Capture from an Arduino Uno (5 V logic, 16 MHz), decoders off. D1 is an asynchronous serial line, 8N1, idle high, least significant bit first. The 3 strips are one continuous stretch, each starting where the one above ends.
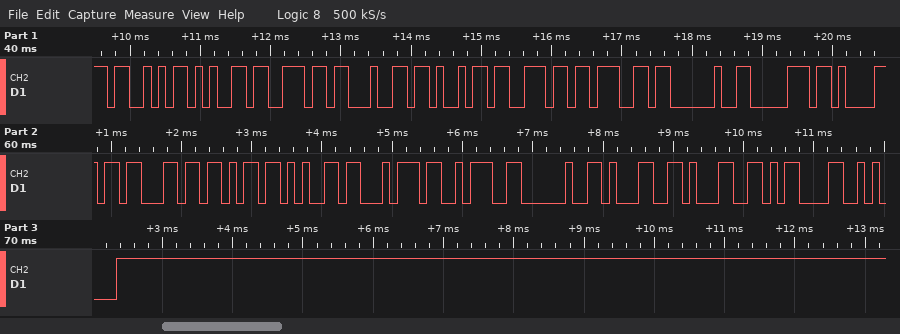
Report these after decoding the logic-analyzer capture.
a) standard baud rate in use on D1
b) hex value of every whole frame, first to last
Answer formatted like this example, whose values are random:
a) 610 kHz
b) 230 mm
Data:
a) 9600 baud
b) 53 65 6E 64 69 6E 67 20 70 61 63 6B 65 74 3A 20 31 31 0D 0A
